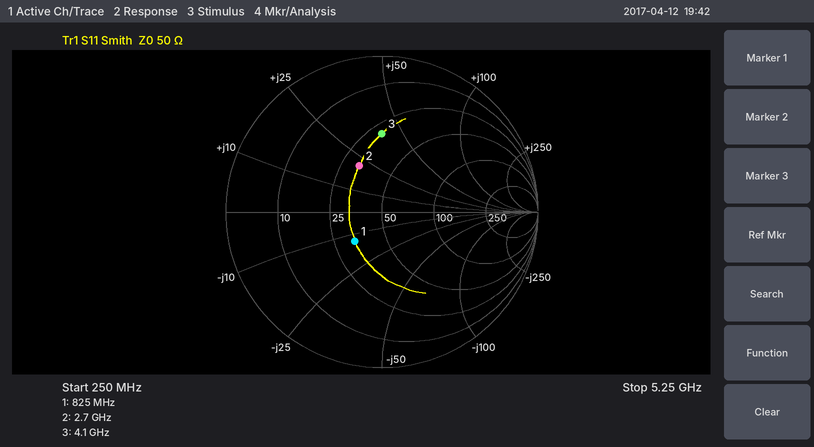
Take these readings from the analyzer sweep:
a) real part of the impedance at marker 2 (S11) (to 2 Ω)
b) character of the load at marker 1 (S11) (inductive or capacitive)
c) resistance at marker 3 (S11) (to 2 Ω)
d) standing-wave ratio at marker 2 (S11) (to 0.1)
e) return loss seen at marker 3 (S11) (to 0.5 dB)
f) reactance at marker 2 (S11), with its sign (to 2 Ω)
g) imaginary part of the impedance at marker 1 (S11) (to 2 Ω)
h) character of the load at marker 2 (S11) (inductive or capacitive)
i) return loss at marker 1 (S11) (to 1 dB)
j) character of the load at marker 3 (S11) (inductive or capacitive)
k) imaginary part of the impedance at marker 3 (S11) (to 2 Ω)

32 Ω
capacitive
30 Ω
2.0
6.0 dB
+22 Ω
-14 Ω
inductive
12 dB
inductive
+40 Ω
